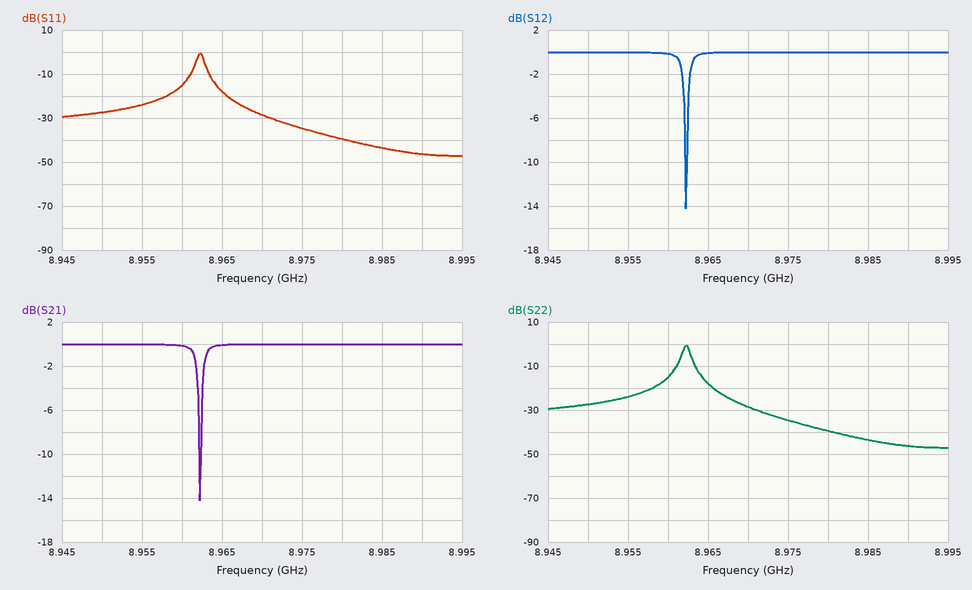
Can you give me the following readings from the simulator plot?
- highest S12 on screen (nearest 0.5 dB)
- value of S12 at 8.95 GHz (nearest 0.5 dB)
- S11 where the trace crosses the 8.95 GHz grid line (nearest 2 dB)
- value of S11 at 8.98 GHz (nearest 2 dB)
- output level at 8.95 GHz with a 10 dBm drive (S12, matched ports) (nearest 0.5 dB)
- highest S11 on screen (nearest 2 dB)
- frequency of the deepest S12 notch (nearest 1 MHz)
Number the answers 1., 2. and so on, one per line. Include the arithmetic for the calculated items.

1. 0.0 dB
2. 0.0 dB
3. -28 dB
4. -40 dB
5. 10 dBm + (0.0 dB) = 10.0 dBm
6. 0 dB
7. 8.962 GHz
